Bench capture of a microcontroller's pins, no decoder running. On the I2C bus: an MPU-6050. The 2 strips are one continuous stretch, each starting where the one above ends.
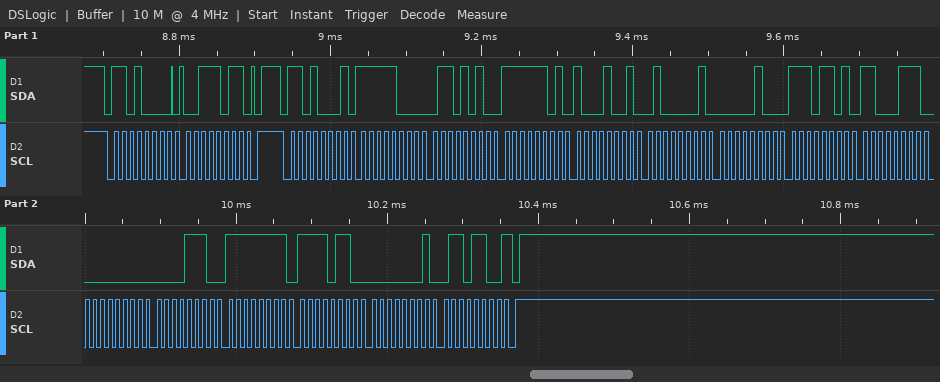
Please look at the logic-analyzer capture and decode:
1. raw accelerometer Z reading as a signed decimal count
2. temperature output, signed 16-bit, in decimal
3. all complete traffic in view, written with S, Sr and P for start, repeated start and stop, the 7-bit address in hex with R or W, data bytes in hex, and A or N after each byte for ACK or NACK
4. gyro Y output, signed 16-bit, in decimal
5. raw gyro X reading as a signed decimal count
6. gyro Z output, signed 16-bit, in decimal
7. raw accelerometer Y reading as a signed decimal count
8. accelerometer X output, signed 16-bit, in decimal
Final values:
16644
-4665
S 68W A 3B A P S 68R A F8 A 6A A FD A 89 A 41 A 04 A ED A C7 A 00 A 0E A FF A F6 A 01 A 6C N P
-10
14
364
-631
-1942
